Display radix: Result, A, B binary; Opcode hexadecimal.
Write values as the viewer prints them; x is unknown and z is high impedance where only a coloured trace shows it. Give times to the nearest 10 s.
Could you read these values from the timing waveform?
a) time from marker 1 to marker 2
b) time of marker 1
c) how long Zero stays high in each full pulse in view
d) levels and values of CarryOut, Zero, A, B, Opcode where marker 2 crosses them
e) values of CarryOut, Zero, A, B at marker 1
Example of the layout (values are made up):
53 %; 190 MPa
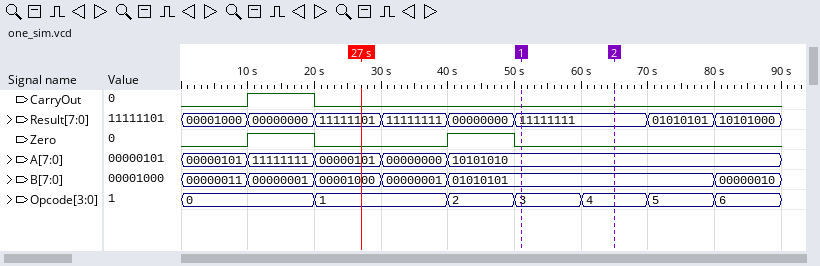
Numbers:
10 s; 50 s; 10 s, 10 s; CarryOut=0, Zero=0, A=10101010, B=01010101, Opcode=4; CarryOut=0, Zero=0, A=10101010, B=01010101
